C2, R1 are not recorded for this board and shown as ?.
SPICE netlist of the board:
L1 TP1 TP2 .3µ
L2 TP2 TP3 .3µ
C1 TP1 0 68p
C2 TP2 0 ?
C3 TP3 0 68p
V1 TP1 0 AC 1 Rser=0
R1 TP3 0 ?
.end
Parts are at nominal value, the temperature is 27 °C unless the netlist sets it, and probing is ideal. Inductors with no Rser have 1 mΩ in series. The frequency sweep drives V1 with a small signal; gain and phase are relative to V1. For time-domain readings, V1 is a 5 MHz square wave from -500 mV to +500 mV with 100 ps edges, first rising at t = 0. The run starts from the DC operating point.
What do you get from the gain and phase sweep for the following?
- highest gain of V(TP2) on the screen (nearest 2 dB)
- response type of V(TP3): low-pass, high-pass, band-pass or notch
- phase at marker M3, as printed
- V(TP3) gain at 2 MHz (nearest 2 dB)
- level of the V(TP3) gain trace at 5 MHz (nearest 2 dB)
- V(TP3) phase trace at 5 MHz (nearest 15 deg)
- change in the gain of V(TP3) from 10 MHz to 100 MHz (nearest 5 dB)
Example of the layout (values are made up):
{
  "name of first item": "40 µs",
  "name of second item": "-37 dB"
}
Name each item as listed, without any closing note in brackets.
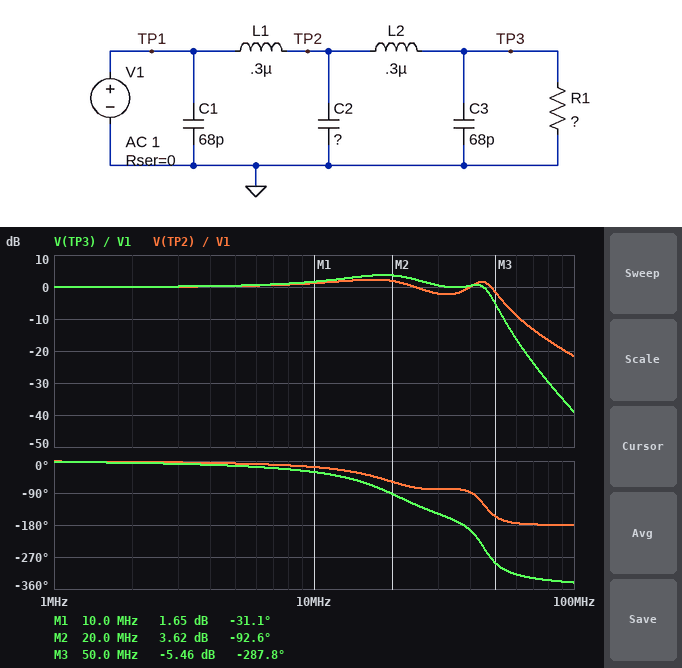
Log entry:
{
  "highest gain of V(TP2) on the screen": "2 dB",
  "response type of V(TP3): low-pass, high-pass, band-pass or notch": "low-pass",
  "phase at marker M3, as printed": "-287.8 deg",
  "V(TP3) gain at 2 MHz": "0 dB",
  "level of the V(TP3) gain trace at 5 MHz": "0 dB",
  "V(TP3) phase trace at 5 MHz": "-15 deg",
  "change in the gain of V(TP3) from 10 MHz to 100 MHz": "-40 dB"
}
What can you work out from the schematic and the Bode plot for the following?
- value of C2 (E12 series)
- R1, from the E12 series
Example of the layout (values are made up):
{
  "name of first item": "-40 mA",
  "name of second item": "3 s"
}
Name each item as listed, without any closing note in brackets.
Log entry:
{
  "value of C2": "120 pF",
  "R1, from the E12 series": "82 Ω"
}
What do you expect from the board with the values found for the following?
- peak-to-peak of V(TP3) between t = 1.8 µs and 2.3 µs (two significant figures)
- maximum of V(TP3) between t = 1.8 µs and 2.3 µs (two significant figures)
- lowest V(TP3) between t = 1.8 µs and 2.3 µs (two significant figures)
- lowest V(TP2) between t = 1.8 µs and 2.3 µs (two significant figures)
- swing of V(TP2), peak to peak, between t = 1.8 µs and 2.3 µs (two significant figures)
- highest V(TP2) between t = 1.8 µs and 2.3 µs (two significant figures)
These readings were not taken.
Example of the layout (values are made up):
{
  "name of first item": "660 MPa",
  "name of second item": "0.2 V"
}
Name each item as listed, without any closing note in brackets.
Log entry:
{
  "peak-to-peak of V(TP3) between t = 1.8 µs and 2.3 µs": "1.8 V",
  "maximum of V(TP3) between t = 1.8 µs and 2.3 µs": "890 mV",
  "lowest V(TP3) between t = 1.8 µs and 2.3 µs": "-890 mV",
  "lowest V(TP2) between t = 1.8 µs and 2.3 µs": "-700 mV",
  "swing of V(TP2), peak to peak, between t = 1.8 µs and 2.3 µs": "1.4 V",
  "highest V(TP2) between t = 1.8 µs and 2.3 µs": "700 mV"
}
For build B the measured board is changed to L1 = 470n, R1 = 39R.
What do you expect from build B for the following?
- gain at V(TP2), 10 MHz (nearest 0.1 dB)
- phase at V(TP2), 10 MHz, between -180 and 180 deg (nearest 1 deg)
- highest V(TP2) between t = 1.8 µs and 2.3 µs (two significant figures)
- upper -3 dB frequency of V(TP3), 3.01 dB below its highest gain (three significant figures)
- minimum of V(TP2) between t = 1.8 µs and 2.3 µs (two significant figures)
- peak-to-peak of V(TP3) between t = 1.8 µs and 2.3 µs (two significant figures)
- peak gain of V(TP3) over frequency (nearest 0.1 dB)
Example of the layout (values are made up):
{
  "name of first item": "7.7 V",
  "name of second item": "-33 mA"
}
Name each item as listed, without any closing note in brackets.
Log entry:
{
  "gain at V(TP2), 10 MHz": "-1.8 dB",
  "phase at V(TP2), 10 MHz, between -180 and 180 deg": "-35 deg",
  "highest V(TP2) between t = 1.8 µs and 2.3 µs": "520 mV",
  "upper -3 dB frequency of V(TP3), 3.01 dB below its highest gain": "13.0 MHz",
  "minimum of V(TP2) between t = 1.8 µs and 2.3 µs": "-520 mV",
  "peak-to-peak of V(TP3) between t = 1.8 µs and 2.3 µs": "1.0 V",
  "peak gain of V(TP3) over frequency": "0 dB"
}
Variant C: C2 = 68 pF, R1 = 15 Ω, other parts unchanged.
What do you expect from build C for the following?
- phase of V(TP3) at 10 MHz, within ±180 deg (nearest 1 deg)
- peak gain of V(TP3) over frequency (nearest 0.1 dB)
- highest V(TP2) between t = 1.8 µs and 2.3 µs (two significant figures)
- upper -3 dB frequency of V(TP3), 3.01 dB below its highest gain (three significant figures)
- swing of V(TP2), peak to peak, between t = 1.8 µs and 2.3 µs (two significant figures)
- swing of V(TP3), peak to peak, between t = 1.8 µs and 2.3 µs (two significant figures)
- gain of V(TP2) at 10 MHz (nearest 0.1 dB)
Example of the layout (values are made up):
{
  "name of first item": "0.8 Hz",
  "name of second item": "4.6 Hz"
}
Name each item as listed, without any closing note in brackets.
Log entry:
{
  "phase of V(TP3) at 10 MHz, within ±180 deg": "-72 deg",
  "peak gain of V(TP3) over frequency": "0.1 dB",
  "highest V(TP2) between t = 1.8 µs and 2.3 µs": "590 mV",
  "upper -3 dB frequency of V(TP3), 3.01 dB below its highest gain": "52.0 MHz",
  "swing of V(TP2), peak to peak, between t = 1.8 µs and 2.3 µs": "1.2 V",
  "swing of V(TP3), peak to peak, between t = 1.8 µs and 2.3 µs": "880 mV",
  "gain of V(TP2) at 10 MHz": "-4.2 dB"
}
